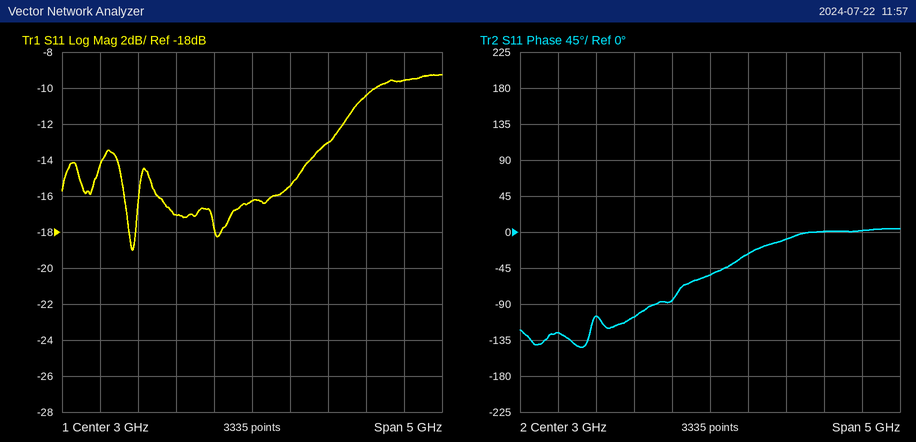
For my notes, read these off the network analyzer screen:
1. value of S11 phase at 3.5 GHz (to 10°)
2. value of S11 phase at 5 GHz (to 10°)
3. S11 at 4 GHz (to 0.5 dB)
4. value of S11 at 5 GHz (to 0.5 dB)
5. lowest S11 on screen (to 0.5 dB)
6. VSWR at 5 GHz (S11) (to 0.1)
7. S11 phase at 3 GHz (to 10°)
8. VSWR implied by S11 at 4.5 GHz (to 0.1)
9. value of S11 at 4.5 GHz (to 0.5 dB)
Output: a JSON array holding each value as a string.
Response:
["-30°", "0°", "-13.0 dB", "-9.5 dB", "-19.0 dB", "2.0", "-50°", "1.9", "-10.5 dB"]
